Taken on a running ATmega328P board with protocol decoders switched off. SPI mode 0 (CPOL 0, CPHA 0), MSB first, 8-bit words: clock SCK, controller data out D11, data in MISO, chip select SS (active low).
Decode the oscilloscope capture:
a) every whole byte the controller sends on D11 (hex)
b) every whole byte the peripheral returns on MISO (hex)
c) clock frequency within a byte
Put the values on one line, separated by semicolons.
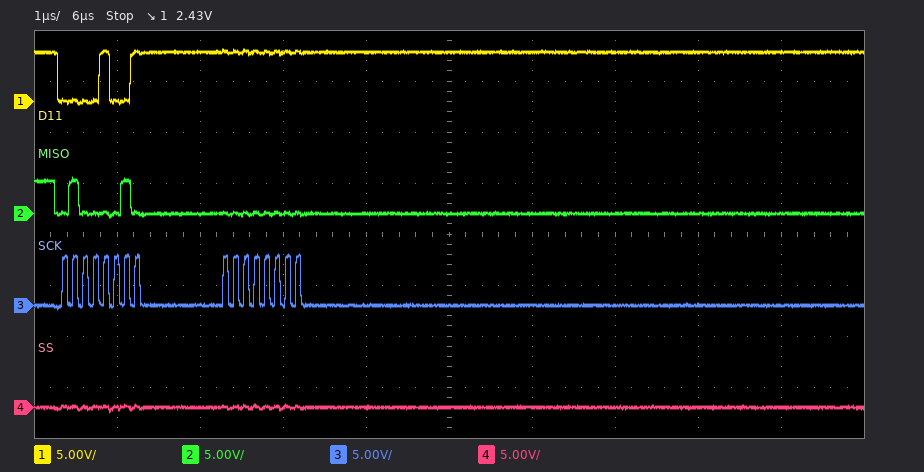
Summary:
0x09 0xFF; 0x42 0x00; 8 MHz
